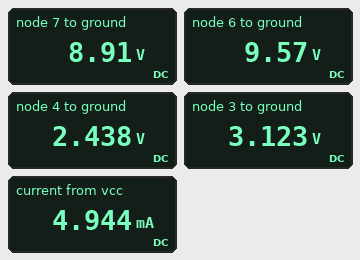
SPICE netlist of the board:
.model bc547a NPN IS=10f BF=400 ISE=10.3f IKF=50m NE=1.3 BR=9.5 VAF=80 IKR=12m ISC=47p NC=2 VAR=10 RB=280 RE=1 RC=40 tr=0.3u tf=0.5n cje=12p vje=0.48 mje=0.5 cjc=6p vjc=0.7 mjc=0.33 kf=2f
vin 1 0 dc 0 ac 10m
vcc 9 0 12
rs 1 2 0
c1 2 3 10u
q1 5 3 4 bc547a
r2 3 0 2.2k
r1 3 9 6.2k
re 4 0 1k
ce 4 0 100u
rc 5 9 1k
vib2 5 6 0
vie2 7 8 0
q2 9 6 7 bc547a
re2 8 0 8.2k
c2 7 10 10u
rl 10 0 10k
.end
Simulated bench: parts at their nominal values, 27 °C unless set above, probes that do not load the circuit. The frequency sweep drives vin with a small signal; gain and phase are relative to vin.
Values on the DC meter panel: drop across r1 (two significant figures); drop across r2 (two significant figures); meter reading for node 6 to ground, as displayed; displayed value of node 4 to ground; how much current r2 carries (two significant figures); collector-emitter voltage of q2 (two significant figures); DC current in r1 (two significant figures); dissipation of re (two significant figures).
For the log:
8.9 V
3.1 V
9.57 V
2.438 V
1.4 mA
3.1 V
1.4 mA
5.9 mW
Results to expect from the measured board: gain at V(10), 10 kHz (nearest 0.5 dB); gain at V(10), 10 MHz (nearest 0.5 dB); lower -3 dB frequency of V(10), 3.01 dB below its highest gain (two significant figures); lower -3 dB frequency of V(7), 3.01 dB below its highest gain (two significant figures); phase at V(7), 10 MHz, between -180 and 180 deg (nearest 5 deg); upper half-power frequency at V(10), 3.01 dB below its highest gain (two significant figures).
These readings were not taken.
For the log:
37.0 dB
22.5 dB
120 Hz
120 Hz
90 deg
1.9 MHz
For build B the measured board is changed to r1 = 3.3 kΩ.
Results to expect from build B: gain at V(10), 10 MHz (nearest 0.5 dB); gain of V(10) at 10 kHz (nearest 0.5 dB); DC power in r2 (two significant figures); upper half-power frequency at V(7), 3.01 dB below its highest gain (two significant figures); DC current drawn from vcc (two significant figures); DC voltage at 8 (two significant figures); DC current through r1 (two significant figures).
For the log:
21.5 dB
40.0 dB
10 mW
1.2 MHz
7.1 mA
7.3 V
2.2 mA
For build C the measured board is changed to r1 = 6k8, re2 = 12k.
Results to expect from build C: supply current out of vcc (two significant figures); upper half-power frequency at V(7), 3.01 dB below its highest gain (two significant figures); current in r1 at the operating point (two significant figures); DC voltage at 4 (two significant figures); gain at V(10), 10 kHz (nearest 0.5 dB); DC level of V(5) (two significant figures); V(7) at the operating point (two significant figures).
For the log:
4.3 mA
2.1 MHz
1.3 mA
2.2 V
36.5 dB
9.8 V
9.1 V
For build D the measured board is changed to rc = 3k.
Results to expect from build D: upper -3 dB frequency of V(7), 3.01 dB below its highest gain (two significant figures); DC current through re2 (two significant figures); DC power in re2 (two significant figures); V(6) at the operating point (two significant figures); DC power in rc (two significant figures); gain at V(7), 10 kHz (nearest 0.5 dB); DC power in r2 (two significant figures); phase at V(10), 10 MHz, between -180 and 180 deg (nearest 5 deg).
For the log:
590 kHz
500 µA
2.0 mW
4.7 V
18 mW
46.0 dB
4.4 mW
85 deg
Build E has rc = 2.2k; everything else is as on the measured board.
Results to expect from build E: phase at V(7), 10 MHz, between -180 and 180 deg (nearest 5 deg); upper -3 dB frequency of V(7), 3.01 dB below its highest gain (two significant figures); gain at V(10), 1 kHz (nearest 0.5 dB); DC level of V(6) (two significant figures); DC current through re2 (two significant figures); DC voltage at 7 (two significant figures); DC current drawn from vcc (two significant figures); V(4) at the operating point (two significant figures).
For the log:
85 deg
910 kHz
43.5 dB
6.7 V
730 µA
6.0 V
4.6 mA
2.4 V
